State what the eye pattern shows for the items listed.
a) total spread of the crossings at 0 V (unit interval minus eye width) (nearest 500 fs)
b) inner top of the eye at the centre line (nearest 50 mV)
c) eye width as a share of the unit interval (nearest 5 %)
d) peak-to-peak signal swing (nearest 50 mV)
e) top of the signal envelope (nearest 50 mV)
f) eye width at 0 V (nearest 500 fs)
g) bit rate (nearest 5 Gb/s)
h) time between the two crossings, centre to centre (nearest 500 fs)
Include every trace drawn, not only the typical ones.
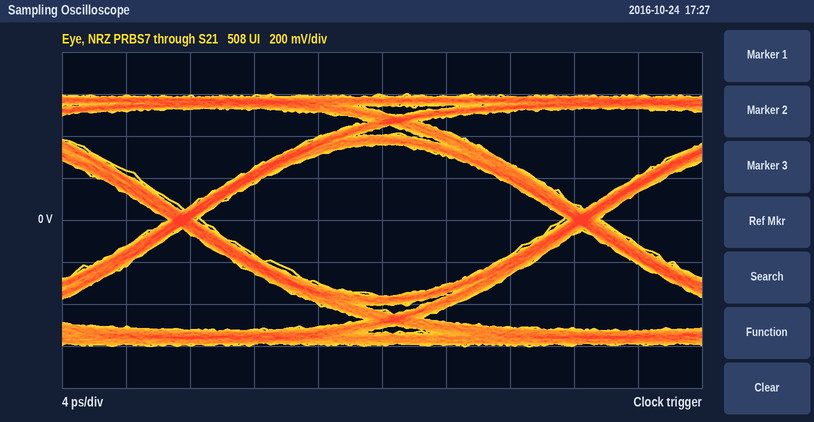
2.5 ps
350 mV
90 %
1.20 V
600 mV
22.5 ps
40 Gb/s
25.0 ps
